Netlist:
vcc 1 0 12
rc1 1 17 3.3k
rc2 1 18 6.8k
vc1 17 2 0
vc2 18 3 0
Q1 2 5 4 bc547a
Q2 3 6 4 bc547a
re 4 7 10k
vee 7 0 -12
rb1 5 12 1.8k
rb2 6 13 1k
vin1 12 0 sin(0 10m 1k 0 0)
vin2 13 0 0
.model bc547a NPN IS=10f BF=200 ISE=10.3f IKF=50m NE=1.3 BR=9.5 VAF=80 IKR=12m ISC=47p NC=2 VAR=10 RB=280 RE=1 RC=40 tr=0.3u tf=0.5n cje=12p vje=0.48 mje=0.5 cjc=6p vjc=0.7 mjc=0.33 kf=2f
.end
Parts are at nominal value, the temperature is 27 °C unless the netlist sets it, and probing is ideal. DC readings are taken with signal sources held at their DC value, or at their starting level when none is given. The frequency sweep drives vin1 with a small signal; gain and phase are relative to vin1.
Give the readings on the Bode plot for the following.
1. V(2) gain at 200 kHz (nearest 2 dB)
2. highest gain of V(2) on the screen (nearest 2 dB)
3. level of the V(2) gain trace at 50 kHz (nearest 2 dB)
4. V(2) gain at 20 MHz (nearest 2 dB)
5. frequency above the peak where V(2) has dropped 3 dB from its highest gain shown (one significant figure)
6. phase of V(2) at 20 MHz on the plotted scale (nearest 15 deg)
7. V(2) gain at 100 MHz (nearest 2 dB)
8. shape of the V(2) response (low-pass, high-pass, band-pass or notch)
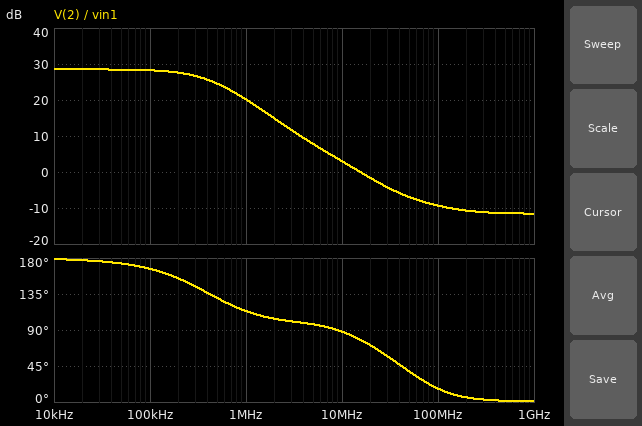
28 dB
28 dB
28 dB
-2 dB
400 kHz
75 deg
-10 dB
low-pass
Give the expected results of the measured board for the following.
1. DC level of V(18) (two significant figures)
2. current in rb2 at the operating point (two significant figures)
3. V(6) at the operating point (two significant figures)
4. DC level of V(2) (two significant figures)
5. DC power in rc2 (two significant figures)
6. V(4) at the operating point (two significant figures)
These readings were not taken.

8.0 V
4.8 µA
-4.8 mV
10 V
2.3 mW
-650 mV
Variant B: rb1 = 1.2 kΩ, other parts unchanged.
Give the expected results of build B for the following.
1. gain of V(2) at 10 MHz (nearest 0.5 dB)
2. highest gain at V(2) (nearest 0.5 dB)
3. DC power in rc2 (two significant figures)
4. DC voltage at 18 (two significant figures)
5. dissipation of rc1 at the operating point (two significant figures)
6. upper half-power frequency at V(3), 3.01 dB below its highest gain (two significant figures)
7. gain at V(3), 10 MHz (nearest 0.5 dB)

4.5 dB
29.0 dB
2.2 mW
8.2 V
1.0 mW
450 kHz
6.0 dB
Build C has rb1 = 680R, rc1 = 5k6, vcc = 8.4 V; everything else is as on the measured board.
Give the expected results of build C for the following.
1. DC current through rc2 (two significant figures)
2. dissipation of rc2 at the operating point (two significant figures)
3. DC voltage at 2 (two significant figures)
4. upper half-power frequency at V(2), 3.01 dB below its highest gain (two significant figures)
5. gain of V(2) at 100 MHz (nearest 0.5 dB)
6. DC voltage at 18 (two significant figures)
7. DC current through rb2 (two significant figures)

550 µA
2.0 mW
5.2 V
380 kHz
-4.5 dB
4.7 V
4.7 µA
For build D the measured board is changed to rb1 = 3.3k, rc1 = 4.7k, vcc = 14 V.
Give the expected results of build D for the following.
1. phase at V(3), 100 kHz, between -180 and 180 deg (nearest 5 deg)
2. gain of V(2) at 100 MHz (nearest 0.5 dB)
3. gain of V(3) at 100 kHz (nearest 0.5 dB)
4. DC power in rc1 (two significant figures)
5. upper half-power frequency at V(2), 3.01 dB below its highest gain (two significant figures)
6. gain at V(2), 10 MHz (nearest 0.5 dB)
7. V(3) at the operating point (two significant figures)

-20 deg
-12.5 dB
33.5 dB
1.1 mW
300 kHz
1.0 dB
9.7 V
